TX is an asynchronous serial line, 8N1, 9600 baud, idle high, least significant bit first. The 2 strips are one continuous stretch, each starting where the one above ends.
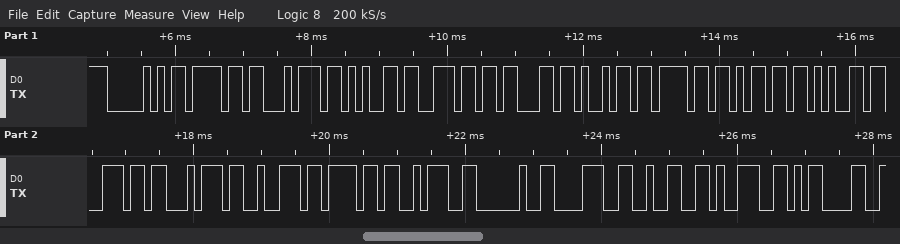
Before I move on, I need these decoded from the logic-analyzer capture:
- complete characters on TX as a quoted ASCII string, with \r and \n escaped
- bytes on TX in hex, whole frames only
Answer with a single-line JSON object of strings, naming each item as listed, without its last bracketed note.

{"complete characters on TX as a quoted ASCII string, with \\r and \\n escaped": "\"Potenciomentro: 829\\r\"", "bytes on TX in hex, whole frames only": "50 6F 74 65 6E 63 69 6F 6D 65 6E 74 72 6F 3A 20 38 32 39 0D"}
